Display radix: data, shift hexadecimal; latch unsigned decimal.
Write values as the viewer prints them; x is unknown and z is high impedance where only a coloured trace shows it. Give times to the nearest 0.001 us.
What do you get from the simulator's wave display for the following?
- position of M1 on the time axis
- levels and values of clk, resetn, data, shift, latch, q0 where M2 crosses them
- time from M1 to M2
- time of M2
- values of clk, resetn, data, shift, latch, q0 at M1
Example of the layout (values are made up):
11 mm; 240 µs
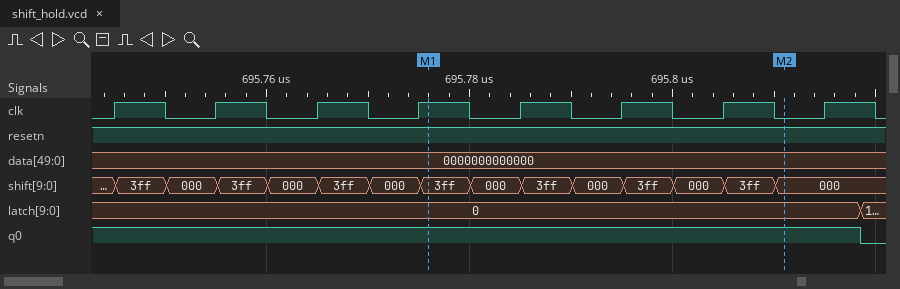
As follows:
695.776 us; clk=0, resetn=1, data=0000000000000, shift=000, latch=0, q0=1; 0.035 us; 695.811 us; clk=1, resetn=1, data=0000000000000, shift=3ff, latch=0, q0=1
